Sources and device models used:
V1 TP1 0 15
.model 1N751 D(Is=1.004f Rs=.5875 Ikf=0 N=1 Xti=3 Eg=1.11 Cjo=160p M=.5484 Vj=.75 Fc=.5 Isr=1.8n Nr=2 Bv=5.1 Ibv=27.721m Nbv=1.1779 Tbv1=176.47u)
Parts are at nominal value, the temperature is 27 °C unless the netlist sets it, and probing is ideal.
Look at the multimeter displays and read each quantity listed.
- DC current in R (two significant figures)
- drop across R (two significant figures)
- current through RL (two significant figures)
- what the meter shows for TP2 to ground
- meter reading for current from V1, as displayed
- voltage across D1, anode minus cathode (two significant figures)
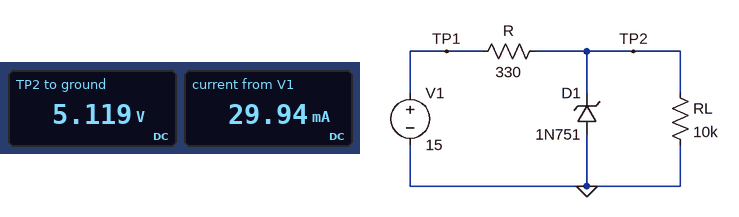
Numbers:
30 mA
9.9 V
510 µA
5.119 V
29.94 mA
-5.1 V
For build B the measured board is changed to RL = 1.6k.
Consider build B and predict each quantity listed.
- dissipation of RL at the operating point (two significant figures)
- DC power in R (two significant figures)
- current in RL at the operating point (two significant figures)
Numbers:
16 mW
300 mW
3.2 mA
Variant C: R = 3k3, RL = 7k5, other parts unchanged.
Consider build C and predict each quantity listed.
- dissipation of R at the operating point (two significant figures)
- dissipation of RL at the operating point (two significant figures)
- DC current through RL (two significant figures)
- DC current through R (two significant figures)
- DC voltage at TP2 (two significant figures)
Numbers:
30 mW
3.4 mW
670 µA
3.0 mA
5.0 V
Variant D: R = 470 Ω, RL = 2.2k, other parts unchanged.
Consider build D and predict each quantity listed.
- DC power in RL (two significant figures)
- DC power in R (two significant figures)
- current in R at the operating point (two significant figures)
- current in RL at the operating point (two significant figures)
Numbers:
12 mW
210 mW
21 mA
2.3 mA
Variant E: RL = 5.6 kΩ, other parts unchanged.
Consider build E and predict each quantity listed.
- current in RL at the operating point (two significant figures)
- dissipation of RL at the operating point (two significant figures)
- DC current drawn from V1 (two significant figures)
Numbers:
910 µA
4.7 mW
30 mA
